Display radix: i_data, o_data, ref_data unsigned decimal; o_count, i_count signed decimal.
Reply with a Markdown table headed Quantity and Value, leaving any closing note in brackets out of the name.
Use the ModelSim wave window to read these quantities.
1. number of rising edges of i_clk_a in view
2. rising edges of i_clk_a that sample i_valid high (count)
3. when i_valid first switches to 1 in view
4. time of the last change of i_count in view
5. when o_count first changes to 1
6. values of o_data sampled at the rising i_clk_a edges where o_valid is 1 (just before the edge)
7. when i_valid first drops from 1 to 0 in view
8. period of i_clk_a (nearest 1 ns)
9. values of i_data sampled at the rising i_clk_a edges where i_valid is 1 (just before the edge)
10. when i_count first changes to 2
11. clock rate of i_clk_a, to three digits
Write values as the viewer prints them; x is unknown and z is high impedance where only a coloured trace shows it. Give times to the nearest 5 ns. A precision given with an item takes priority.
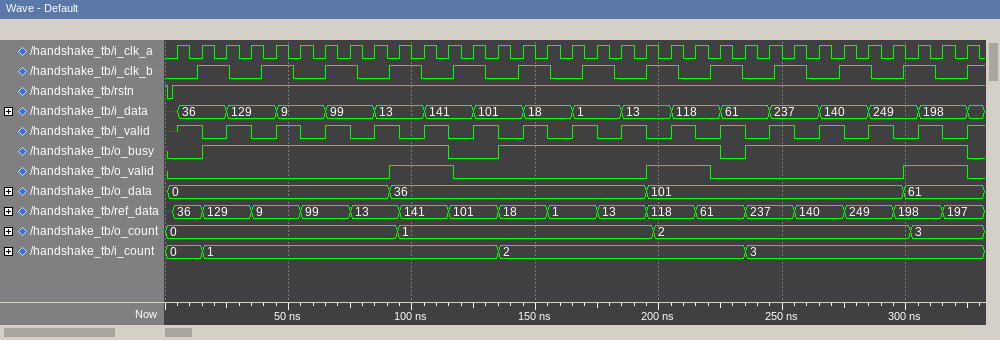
| Quantity | Value |
|---|---|
| number of rising edges of i_clk_a in view | 33 |
| rising edges of i_clk_a that sample i_valid high | 16 |
| when i_valid first switches to 1 in view | 5 ns |
| time of the last change of i_count in view | 235 ns |
| when o_count first changes to 1 | 95 ns |
| values of o_data sampled at the rising i_clk_a edges where o_valid is 1 | 36, 36, 36, 101, 101, 61, 61, 61 |
| when i_valid first drops from 1 to 0 in view | 15 ns |
| period of i_clk_a | 10 ns |
| values of i_data sampled at the rising i_clk_a edges where i_valid is 1 | 36, 129, 9, 99, 13, 141, 101, 18, 1, 13, 118, 61, 237, 140, 249, 198 |
| when i_count first changes to 2 | 135 ns |
| clock rate of i_clk_a, to three digits | 100 MHz |
